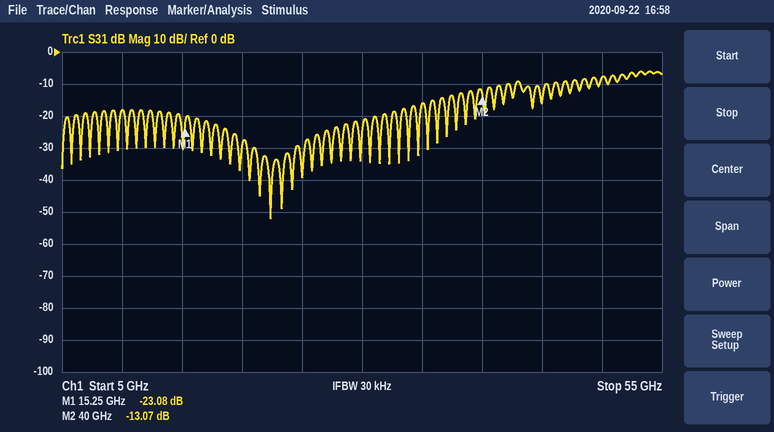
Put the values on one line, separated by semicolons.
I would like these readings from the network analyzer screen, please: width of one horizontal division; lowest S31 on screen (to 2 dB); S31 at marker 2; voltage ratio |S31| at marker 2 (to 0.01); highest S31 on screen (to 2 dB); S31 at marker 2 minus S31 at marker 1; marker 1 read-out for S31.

5 GHz; -52 dB; -13.07 dB; 0.22; -6 dB; 10.01 dB; -23.08 dB
